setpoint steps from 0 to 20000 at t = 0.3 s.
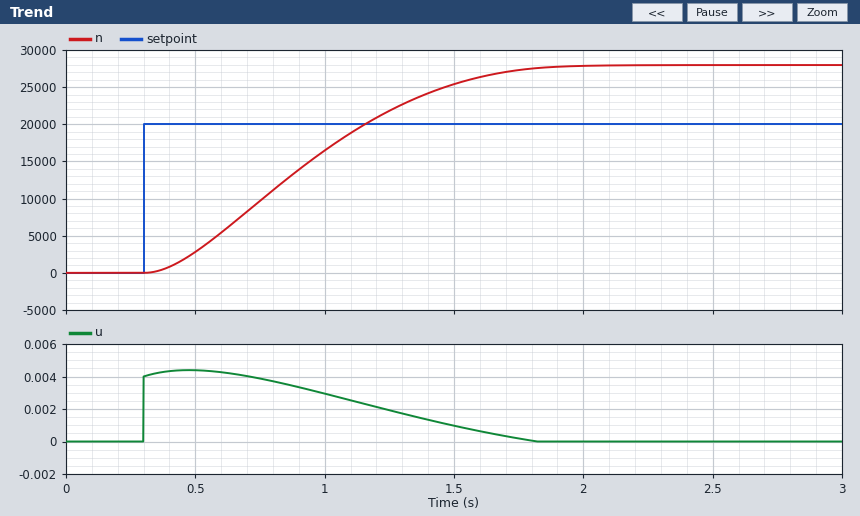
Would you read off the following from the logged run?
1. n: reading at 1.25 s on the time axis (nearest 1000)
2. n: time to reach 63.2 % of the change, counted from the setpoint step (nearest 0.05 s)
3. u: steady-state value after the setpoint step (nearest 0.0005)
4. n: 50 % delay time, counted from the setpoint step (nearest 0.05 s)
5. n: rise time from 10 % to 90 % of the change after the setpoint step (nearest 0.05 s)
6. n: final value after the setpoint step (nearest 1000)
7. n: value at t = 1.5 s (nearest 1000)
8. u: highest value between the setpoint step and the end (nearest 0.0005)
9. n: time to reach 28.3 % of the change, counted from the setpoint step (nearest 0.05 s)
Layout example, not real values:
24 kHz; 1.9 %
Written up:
22000; 0.75 s; 0.0000; 0.60 s; 1.00 s; 28000; 25000; 0.0045; 0.40 s
